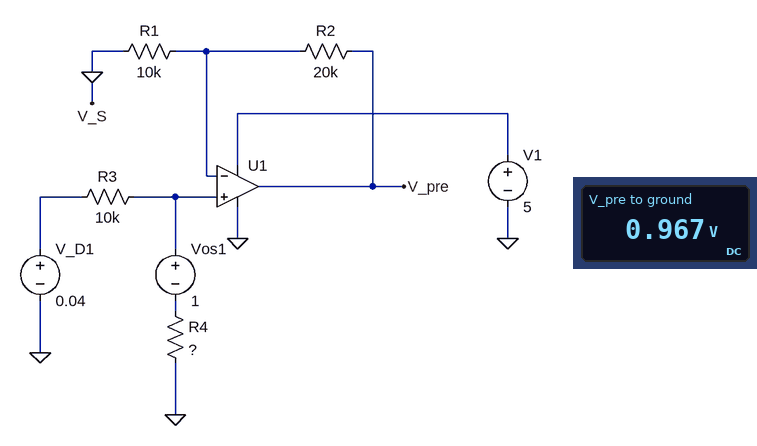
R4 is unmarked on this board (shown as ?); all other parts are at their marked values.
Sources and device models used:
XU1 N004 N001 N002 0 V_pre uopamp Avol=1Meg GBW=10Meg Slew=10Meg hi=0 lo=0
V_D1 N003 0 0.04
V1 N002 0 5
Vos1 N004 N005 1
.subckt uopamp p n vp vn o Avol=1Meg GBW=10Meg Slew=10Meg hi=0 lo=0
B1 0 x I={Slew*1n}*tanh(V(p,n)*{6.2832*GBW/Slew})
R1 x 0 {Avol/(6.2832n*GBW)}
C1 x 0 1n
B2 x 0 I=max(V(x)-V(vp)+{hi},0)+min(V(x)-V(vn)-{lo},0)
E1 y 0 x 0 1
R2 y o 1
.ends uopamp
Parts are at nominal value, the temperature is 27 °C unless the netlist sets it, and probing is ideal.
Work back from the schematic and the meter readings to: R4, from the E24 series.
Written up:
24 kΩ
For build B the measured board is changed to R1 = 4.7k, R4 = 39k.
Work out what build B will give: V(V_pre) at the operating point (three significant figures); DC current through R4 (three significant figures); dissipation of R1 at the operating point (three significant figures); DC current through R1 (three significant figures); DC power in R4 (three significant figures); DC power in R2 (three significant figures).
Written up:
1.24 V
19.6 µA
11.8 µW
50.2 µA
15.0 µW
50.4 µW
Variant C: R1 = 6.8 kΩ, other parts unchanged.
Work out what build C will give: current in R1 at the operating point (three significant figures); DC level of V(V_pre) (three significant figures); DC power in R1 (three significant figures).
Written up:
47.4 µA
1.27 V
15.3 µW
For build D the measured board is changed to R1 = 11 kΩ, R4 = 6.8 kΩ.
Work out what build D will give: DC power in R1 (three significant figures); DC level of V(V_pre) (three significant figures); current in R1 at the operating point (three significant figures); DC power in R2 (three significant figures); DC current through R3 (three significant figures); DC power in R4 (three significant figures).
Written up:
34.0 µW
1.72 V
55.6 µA
61.8 µW
57.1 µA
22.2 µW
